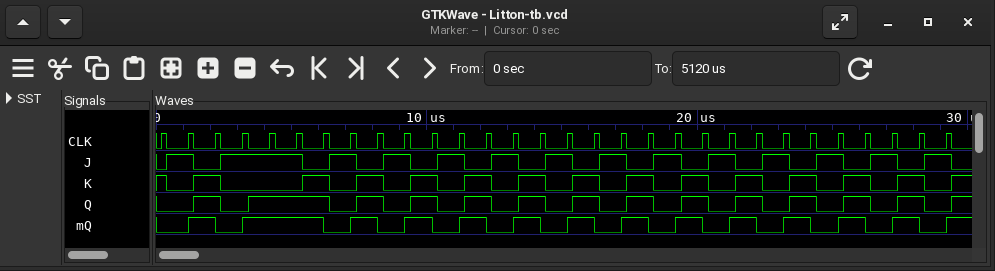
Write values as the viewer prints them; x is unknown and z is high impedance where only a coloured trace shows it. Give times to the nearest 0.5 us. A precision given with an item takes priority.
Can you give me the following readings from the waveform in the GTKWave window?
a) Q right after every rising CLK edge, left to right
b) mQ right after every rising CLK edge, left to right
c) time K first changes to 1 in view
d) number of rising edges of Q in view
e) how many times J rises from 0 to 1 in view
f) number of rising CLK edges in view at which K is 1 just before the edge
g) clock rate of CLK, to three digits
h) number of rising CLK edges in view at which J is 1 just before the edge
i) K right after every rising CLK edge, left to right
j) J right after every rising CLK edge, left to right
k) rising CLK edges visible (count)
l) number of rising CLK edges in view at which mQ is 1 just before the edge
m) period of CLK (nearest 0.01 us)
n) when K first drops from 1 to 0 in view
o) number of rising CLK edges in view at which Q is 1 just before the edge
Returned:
0 0 1 0 1 1 1 0 1 0 1 0 1 0 1 0 1 0 1 0 1 0 1 0 1 0 1 0 1 0
0 1 0 1 1 1 0 1 0 1 0 1 0 1 0 1 0 1 0 1 0 1 0 1 0 1 0 1 0 1
1.5 us
14
14
14
1.00 MHz
16
1 0 1 0 0 0 1 0 1 0 1 0 1 0 1 0 1 0 1 0 1 0 1 0 1 0 1 0 1 0
0 1 0 1 1 1 0 1 0 1 0 1 0 1 0 1 0 1 0 1 0 1 0 1 0 1 0 1 0 1
30
15
1 us
0.5 us
15
